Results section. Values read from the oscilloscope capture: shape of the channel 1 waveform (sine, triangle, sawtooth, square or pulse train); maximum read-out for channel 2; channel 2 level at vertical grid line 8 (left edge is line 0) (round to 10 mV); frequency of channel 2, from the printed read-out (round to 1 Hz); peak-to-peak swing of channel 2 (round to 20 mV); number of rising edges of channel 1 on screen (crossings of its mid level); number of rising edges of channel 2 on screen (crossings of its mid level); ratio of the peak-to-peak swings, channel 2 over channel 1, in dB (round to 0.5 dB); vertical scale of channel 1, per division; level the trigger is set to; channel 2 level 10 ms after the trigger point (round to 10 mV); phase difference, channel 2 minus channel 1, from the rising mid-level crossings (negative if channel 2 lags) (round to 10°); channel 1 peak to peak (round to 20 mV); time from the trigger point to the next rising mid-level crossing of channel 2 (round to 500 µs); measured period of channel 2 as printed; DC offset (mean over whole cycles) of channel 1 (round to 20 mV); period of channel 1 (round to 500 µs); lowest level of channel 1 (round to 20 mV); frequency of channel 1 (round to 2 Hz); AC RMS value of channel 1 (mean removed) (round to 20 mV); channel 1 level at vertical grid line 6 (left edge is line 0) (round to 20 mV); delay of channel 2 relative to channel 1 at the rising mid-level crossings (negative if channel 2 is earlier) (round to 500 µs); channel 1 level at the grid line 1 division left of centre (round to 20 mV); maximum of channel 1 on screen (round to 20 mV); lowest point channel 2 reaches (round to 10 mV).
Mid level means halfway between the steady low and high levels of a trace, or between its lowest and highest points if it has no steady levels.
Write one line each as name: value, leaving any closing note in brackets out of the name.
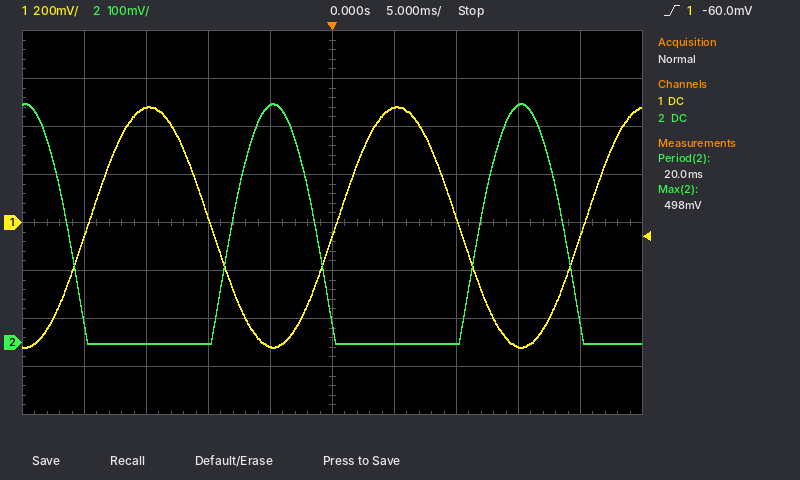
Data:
shape of the channel 1 waveform: sine
maximum read-out for channel 2: 498 mV
channel 2 level at vertical grid line 8 (left edge is line 0): 490 mV
frequency of channel 2, from the printed read-out: 50 Hz
peak-to-peak swing of channel 2: 500 mV
number of rising edges of channel 1 on screen: 3
number of rising edges of channel 2 on screen: 2
ratio of the peak-to-peak swings, channel 2 over channel 1, in dB: -6.0 dB
vertical scale of channel 1, per division: 200 mV
level the trigger is set to: -60.0 mV
channel 2 level 10 ms after the trigger point: 0 mV
phase difference, channel 2 minus channel 1, from the rising mid-level crossings (negative if channel 2 lags): +150°
channel 1 peak to peak: 1.00 V
time from the trigger point to the next rising mid-level crossing of channel 2: 12.0 ms
measured period of channel 2 as printed: 20.0 ms
DC offset (mean over whole cycles) of channel 1: -20 mV
period of channel 1: 20.0 ms
lowest level of channel 1: -520 mV
frequency of channel 1: 50 Hz
AC RMS value of channel 1 (mean removed): 360 mV
channel 1 level at vertical grid line 6 (left edge is line 0): 480 mV
delay of channel 2 relative to channel 1 at the rising mid-level crossings (negative if channel 2 is earlier): -8.5 ms
channel 1 level at the grid line 1 division left of centre: -520 mV
maximum of channel 1 on screen: 480 mV
lowest point channel 2 reaches: 0 mV
